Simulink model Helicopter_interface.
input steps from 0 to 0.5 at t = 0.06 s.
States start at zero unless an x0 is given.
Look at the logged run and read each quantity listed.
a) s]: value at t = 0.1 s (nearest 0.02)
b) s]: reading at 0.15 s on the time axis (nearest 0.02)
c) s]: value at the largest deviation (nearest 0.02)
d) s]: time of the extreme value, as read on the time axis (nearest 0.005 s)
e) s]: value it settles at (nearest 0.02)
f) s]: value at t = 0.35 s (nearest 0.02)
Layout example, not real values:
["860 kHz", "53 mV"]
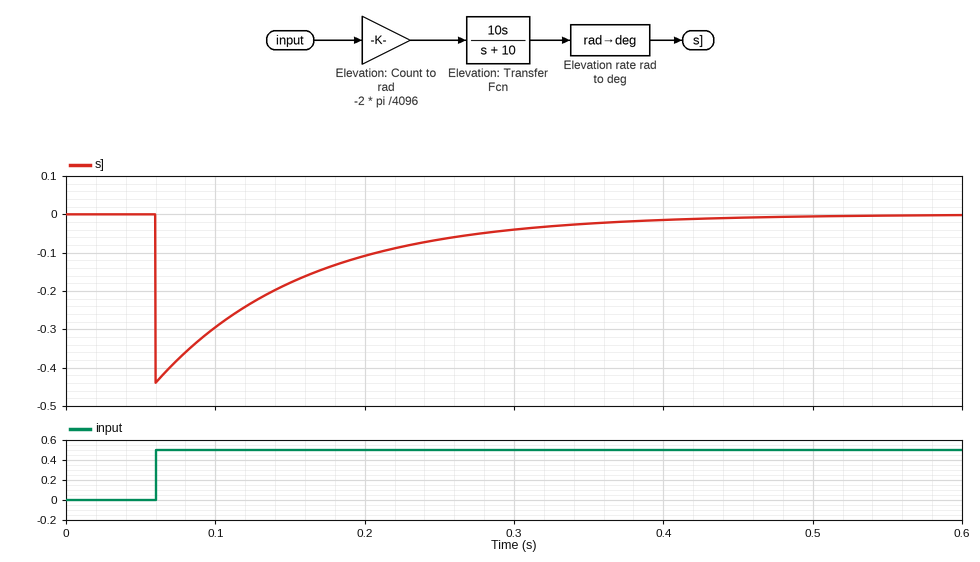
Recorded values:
["-0.30", "-0.18", "-0.44", "0.060 s", "0.00", "-0.02"]
